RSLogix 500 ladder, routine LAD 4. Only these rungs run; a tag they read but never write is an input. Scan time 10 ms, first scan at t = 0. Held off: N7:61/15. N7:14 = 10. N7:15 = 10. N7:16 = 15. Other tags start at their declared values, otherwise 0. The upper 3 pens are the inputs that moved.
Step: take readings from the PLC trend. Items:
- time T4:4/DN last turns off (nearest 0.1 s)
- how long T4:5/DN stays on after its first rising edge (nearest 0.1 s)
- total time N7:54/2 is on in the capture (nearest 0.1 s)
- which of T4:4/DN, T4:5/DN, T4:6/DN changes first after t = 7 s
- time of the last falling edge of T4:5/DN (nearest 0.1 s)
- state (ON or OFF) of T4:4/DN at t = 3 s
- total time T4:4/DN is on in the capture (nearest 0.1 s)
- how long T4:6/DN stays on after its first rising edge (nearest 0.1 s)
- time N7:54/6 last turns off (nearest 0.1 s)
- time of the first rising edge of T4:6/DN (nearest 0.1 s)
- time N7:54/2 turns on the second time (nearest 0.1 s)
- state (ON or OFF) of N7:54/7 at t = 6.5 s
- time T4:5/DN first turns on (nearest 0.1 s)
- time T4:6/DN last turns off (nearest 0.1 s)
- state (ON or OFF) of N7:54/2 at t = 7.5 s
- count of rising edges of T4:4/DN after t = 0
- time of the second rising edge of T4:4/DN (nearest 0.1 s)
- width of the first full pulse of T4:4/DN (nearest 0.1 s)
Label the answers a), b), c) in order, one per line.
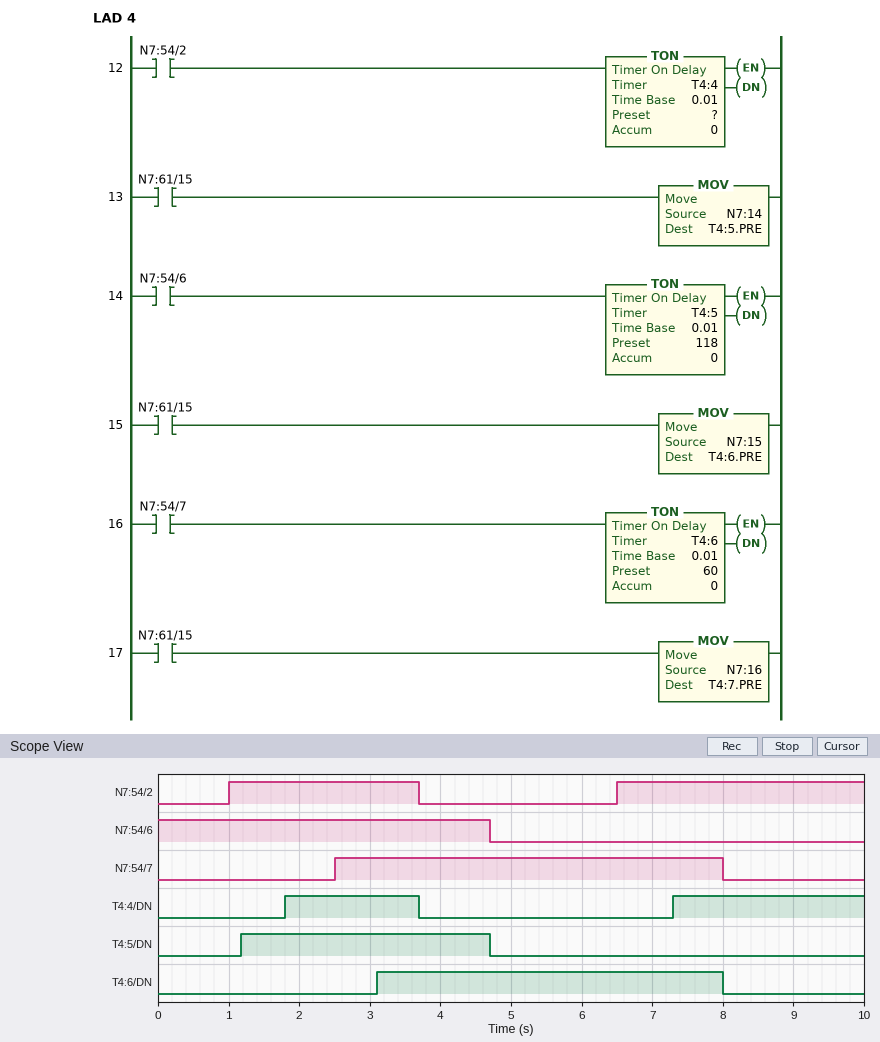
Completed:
a) 3.7 s
b) 3.5 s
c) 6.2 s
d) T4:4/DN
e) 4.7 s
f) ON
g) 4.6 s
h) 4.9 s
i) 4.7 s
j) 3.1 s
k) 6.5 s
l) ON
m) 1.2 s
n) 8.0 s
o) ON
p) 2
q) 7.3 s
r) 1.9 s
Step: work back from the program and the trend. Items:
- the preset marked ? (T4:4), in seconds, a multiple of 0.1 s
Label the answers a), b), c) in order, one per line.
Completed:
a) 0.8 s
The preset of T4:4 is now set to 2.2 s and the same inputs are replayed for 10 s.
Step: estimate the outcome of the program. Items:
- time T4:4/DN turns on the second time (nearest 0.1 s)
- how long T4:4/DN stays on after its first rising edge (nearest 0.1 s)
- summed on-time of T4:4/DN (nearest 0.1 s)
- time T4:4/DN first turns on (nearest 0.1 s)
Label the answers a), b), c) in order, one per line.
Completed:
a) 8.7 s
b) 0.5 s
c) 1.8 s
d) 3.2 s
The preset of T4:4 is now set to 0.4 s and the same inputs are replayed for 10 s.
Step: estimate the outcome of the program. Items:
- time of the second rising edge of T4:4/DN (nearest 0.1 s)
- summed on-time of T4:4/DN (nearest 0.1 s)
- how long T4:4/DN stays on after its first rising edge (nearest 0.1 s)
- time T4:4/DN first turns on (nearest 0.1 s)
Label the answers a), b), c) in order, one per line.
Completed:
a) 6.9 s
b) 5.4 s
c) 2.3 s
d) 1.4 s
